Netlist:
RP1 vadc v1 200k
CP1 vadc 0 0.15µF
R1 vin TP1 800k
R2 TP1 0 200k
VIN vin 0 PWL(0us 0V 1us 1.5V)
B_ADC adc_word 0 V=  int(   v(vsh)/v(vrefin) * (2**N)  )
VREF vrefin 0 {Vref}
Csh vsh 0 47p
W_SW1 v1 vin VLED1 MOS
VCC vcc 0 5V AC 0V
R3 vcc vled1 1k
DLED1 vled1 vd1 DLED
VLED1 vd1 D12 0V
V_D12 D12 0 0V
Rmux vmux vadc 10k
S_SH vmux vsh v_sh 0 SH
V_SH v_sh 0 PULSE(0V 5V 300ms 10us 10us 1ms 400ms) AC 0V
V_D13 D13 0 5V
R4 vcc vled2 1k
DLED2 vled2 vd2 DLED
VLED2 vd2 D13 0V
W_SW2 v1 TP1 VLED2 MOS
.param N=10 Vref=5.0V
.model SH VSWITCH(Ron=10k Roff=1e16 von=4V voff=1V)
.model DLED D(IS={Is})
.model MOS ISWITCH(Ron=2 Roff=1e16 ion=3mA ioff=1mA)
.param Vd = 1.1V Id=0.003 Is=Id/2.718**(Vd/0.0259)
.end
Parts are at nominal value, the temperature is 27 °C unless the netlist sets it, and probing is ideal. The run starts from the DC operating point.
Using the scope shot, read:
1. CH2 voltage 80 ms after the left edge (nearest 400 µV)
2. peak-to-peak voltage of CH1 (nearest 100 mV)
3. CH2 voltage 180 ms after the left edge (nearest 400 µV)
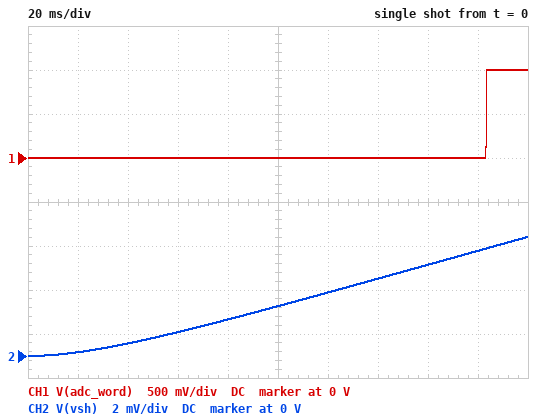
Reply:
1.6 mV
1.0 V
4.8 mV
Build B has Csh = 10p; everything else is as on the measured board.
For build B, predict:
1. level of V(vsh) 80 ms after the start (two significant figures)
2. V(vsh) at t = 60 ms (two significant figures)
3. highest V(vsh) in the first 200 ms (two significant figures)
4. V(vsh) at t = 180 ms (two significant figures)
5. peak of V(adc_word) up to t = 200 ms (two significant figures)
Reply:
7.8 mV
5.1 mV
25 mV
22 mV
5.0 V
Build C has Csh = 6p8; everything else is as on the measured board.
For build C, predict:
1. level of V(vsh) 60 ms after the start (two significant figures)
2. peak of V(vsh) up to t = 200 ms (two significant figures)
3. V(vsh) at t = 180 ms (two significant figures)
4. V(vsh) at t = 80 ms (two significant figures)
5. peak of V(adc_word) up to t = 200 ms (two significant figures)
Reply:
7.5 mV
37 mV
33 mV
11 mV
7.0 V
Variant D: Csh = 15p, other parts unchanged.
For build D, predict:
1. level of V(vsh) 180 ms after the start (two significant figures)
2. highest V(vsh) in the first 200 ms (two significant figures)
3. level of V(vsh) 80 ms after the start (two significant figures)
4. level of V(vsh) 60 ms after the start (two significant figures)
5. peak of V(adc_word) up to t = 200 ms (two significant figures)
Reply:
15 mV
17 mV
5.2 mV
3.4 mV
3.0 V
